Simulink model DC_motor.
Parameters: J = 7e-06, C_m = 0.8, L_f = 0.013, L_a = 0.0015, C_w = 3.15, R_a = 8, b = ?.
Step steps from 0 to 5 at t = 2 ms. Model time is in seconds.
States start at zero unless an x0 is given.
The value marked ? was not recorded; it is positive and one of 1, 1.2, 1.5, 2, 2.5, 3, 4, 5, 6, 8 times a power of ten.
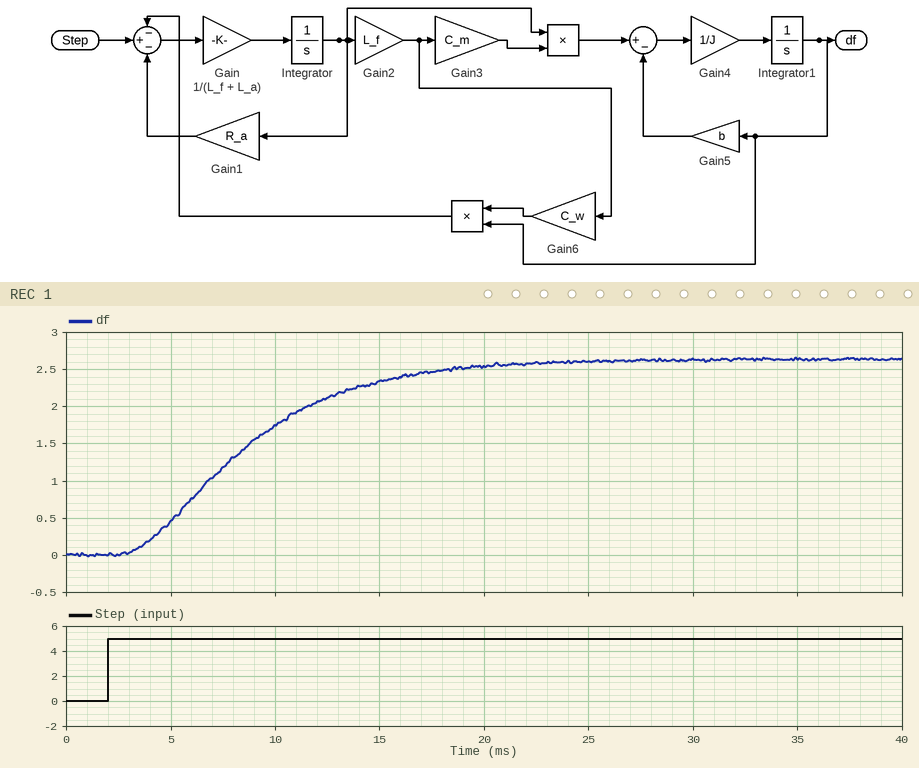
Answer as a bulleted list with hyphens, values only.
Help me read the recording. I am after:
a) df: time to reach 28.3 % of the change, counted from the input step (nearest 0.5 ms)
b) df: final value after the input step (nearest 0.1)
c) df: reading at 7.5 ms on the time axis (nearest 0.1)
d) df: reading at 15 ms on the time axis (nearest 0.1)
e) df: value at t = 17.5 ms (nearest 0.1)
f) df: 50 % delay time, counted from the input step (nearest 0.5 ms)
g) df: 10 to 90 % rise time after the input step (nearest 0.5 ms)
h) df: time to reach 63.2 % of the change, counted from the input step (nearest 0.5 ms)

- 4.0 ms
- 2.6
- 1.2
- 2.3
- 2.5
- 6.0 ms
- 11.5 ms
- 7.5 ms
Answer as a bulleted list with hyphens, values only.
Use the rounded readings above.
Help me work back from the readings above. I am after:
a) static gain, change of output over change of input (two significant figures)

- 0.52
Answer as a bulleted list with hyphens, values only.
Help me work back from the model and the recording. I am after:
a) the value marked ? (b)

- 0.0015
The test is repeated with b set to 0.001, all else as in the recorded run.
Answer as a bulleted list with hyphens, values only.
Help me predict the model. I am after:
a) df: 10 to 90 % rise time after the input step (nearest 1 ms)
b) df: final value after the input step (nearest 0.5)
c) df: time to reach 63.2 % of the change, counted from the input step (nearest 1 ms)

- 16 ms
- 4.0
- 10 ms
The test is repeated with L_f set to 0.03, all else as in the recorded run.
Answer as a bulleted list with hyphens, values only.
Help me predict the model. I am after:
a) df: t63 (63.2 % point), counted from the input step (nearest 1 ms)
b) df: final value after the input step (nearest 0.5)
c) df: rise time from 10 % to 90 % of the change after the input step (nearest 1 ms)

- 10 ms
- 5.5
- 13 ms
